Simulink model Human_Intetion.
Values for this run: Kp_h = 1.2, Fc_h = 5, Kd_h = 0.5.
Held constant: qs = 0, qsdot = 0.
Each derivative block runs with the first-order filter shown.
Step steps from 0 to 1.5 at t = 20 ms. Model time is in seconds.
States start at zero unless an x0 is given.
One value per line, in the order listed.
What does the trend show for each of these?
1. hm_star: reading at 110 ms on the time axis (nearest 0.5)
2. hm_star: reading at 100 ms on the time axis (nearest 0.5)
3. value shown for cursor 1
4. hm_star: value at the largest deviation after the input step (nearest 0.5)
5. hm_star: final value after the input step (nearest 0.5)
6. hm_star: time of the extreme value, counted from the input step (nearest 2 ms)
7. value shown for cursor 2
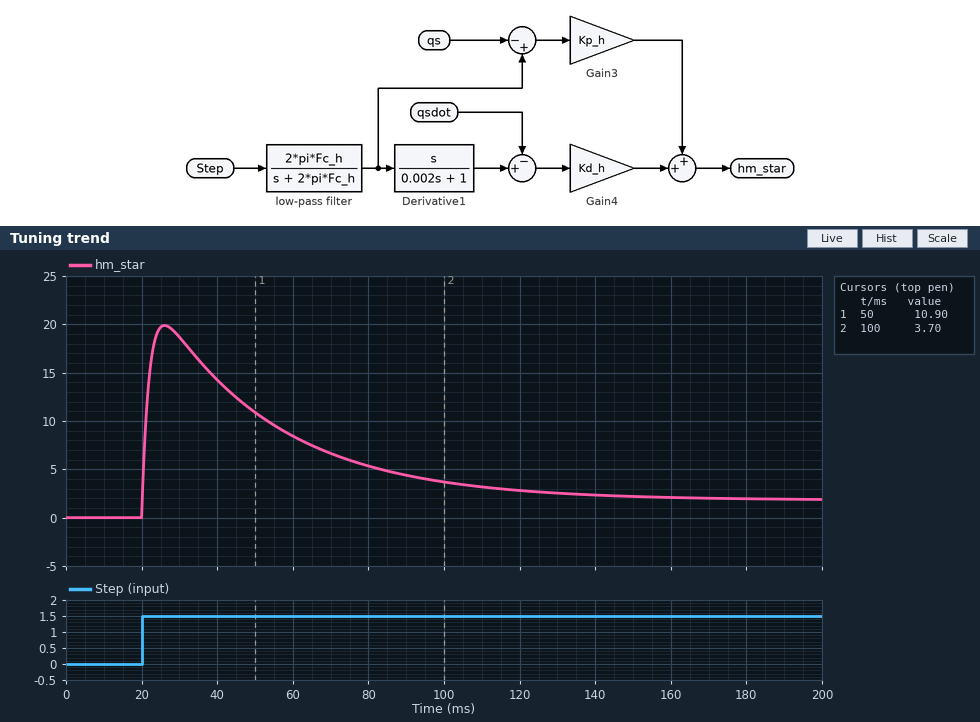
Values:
3.0
3.5
10.90
20.0
2.0
6 ms
3.70
